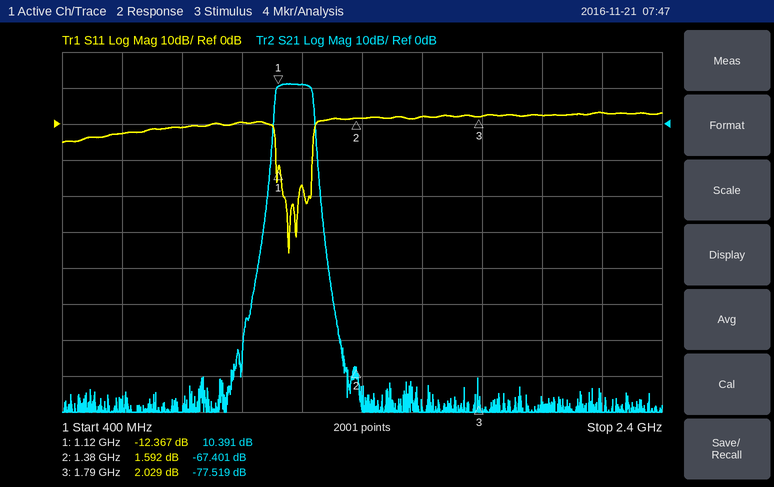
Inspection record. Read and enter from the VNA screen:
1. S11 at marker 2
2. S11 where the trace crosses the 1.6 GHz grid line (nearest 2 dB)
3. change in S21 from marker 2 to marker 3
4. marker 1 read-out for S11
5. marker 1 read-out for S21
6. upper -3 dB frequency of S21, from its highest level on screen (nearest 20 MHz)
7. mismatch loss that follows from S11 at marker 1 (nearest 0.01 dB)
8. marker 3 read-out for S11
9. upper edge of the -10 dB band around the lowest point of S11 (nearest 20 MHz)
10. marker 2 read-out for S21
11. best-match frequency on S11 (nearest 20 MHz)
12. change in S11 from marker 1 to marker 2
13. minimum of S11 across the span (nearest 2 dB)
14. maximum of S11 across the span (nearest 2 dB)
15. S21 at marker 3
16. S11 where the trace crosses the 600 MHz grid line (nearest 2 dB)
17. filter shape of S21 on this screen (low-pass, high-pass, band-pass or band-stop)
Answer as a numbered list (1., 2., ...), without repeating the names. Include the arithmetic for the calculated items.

1. 1.592 dB
2. 2 dB
3. -77.519 − (-67.401) = -10.118 dB
4. -12.367 dB
5. 10.391 dB
6. 1.24 GHz
7. −10 log10(1 − 10^(-12.367/10)) ≈ 0.26 dB
8. 2.029 dB
9. 1.24 GHz
10. -67.401 dB
11. 1.16 GHz
12. 1.592 − (-12.367) = 13.959 dB
13. -36 dB
14. 4 dB
15. -77.519 dB
16. -2 dB
17. band-pass
